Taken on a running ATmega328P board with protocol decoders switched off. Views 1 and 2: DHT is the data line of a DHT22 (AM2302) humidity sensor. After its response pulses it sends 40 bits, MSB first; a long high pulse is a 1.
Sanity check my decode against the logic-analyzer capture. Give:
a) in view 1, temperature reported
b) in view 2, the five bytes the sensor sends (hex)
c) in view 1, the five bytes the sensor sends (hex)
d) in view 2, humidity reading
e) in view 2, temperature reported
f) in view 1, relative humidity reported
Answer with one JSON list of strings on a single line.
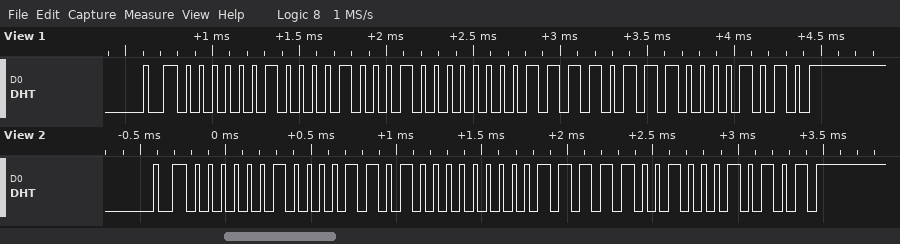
["24.7 °C", "02 1A 00 F9 15", "02 11 00 F7 0A", "53.8 %", "24.9 °C", "52.9 %"]
